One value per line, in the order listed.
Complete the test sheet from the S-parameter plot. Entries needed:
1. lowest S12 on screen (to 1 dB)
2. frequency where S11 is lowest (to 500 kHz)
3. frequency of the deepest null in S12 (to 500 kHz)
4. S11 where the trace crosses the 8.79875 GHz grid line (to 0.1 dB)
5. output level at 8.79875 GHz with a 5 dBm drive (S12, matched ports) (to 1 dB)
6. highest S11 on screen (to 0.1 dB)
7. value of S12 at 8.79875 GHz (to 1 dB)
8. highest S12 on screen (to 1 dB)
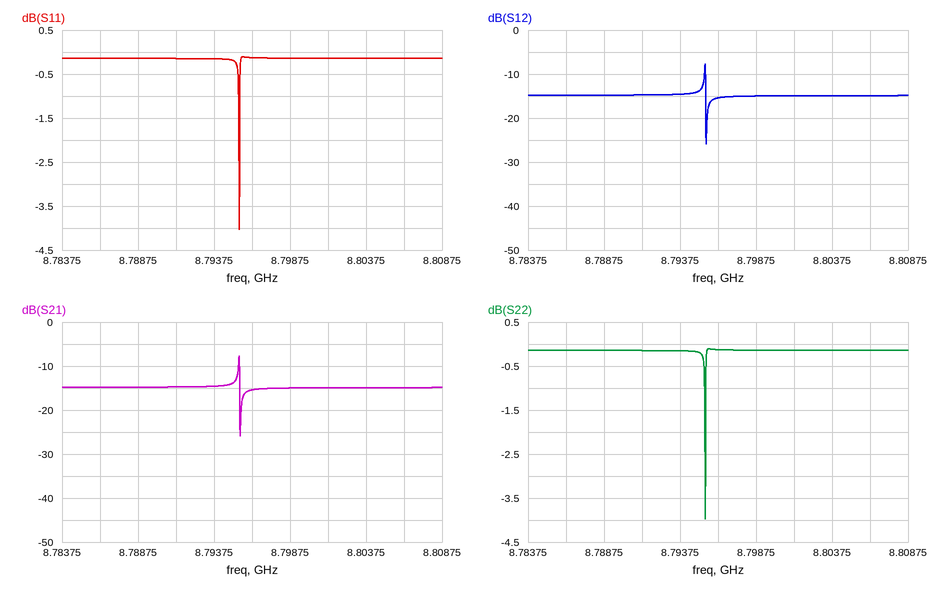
-26 dB
8.7955 GHz
8.7955 GHz
-0.1 dB
-10 dBm
-0.1 dB
-15 dB
-8 dB
